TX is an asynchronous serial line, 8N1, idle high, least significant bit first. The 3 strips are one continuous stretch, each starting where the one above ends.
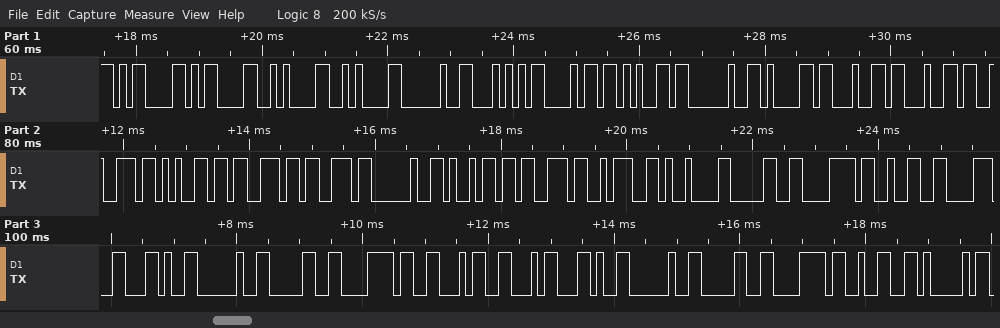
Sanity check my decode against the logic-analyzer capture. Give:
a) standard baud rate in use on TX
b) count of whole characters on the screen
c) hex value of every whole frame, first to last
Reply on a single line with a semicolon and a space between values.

9600 baud; 37; 0D 0D 0A 0A 20 54 68 65 20 61 64 64 72 65 73 73 20 69 73 3A 09 30 78 32 38 2C 20 30 78 46 46 2C 20 30 78 32 41
